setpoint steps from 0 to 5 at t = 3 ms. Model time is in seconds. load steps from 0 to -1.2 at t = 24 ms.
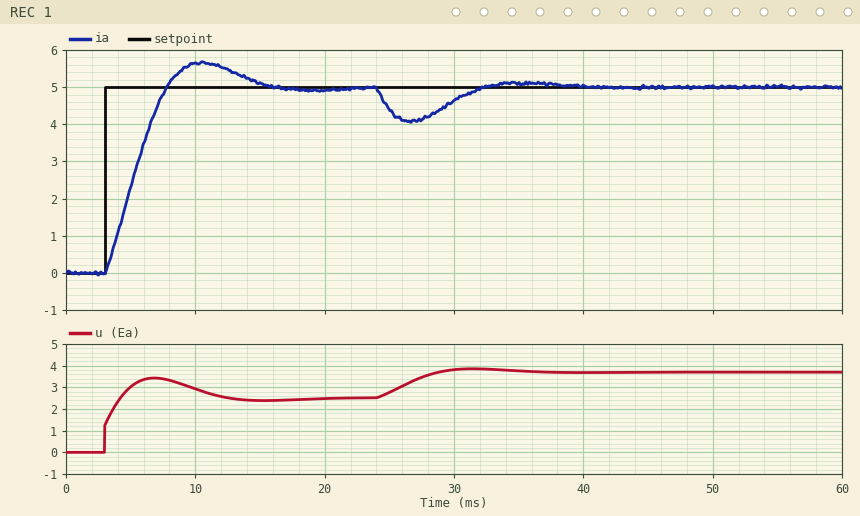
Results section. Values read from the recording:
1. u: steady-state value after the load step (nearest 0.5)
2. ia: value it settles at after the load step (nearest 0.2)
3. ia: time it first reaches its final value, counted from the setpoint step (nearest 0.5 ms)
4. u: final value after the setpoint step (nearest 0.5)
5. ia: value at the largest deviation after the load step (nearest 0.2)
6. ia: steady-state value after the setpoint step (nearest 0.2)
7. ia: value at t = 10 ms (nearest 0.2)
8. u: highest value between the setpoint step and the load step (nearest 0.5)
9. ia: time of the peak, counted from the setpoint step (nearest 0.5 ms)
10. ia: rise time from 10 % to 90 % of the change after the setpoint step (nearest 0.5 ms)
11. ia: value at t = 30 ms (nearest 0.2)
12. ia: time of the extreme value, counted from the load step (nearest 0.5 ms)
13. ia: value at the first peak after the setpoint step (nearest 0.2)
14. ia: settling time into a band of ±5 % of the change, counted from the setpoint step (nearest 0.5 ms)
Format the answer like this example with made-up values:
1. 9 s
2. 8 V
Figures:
1. 3.5
2. 5.0
3. 5.0 ms
4. 2.5
5. 4.0
6. 5.0
7. 5.6
8. 3.5
9. 7.5 ms
10. 3.5 ms
11. 4.6
12. 2.5 ms
13. 5.6
14. 11.0 ms
